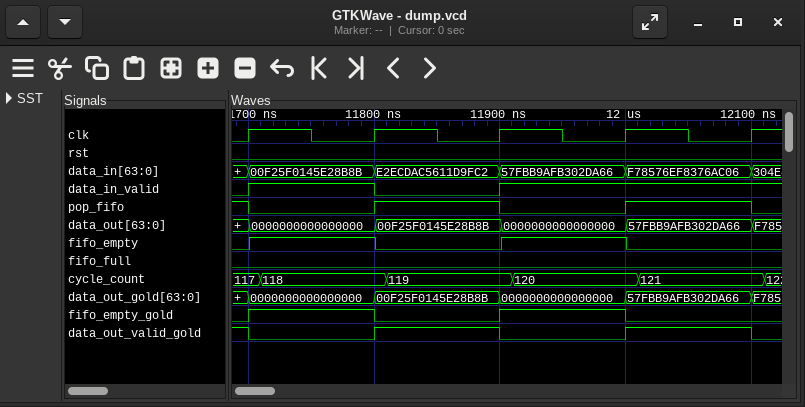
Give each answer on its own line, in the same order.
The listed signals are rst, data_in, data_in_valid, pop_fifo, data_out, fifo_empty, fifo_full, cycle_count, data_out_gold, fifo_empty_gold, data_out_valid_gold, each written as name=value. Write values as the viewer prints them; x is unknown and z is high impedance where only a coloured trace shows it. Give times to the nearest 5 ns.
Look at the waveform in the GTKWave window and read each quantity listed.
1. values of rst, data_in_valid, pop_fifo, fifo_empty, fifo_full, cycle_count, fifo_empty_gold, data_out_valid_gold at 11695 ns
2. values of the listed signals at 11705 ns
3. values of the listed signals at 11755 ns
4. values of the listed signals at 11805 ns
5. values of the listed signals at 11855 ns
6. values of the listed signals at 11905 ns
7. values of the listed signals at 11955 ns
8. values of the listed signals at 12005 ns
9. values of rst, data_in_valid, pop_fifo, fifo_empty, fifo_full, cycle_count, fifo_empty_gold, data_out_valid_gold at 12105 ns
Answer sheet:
rst=0, data_in_valid=0, pop_fifo=1, fifo_empty=0, fifo_full=0, cycle_count=117, fifo_empty_gold=0, data_out_valid_gold=1
rst=0, data_in=00F25F0145E28B8B, data_in_valid=1, pop_fifo=0, data_out=0000000000000000, fifo_empty=1, fifo_full=0, cycle_count=117, data_out_gold=0000000000000000, fifo_empty_gold=1, data_out_valid_gold=0
rst=0, data_in=00F25F0145E28B8B, data_in_valid=1, pop_fifo=0, data_out=0000000000000000, fifo_empty=1, fifo_full=0, cycle_count=118, data_out_gold=0000000000000000, fifo_empty_gold=1, data_out_valid_gold=0
rst=0, data_in=E2ECDAC5611D9FC2, data_in_valid=0, pop_fifo=1, data_out=00F25F0145E28B8B, fifo_empty=0, fifo_full=0, cycle_count=118, data_out_gold=00F25F0145E28B8B, fifo_empty_gold=0, data_out_valid_gold=1
rst=0, data_in=E2ECDAC5611D9FC2, data_in_valid=0, pop_fifo=1, data_out=00F25F0145E28B8B, fifo_empty=0, fifo_full=0, cycle_count=119, data_out_gold=00F25F0145E28B8B, fifo_empty_gold=0, data_out_valid_gold=1
rst=0, data_in=57FBB9AFB302DA66, data_in_valid=1, pop_fifo=0, data_out=0000000000000000, fifo_empty=1, fifo_full=0, cycle_count=119, data_out_gold=0000000000000000, fifo_empty_gold=1, data_out_valid_gold=0
rst=0, data_in=57FBB9AFB302DA66, data_in_valid=1, pop_fifo=0, data_out=0000000000000000, fifo_empty=1, fifo_full=0, cycle_count=120, data_out_gold=0000000000000000, fifo_empty_gold=1, data_out_valid_gold=0
rst=0, data_in=F78576EF8376AC06, data_in_valid=1, pop_fifo=1, data_out=57FBB9AFB302DA66, fifo_empty=0, fifo_full=0, cycle_count=120, data_out_gold=57FBB9AFB302DA66, fifo_empty_gold=0, data_out_valid_gold=1
rst=0, data_in_valid=1, pop_fifo=0, fifo_empty=0, fifo_full=0, cycle_count=121, fifo_empty_gold=0, data_out_valid_gold=0
